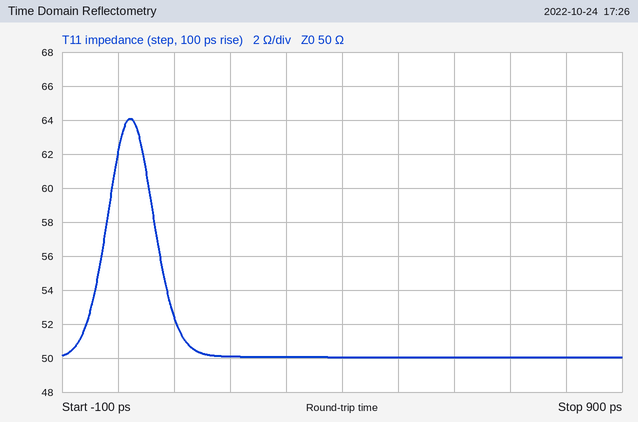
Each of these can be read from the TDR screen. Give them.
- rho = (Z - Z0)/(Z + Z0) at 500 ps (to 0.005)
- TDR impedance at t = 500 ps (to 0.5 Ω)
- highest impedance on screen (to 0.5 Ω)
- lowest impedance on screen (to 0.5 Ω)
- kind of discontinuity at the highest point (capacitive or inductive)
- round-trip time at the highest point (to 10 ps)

0.000
50.0 Ω
64.0 Ω
50.0 Ω
inductive
20 ps
